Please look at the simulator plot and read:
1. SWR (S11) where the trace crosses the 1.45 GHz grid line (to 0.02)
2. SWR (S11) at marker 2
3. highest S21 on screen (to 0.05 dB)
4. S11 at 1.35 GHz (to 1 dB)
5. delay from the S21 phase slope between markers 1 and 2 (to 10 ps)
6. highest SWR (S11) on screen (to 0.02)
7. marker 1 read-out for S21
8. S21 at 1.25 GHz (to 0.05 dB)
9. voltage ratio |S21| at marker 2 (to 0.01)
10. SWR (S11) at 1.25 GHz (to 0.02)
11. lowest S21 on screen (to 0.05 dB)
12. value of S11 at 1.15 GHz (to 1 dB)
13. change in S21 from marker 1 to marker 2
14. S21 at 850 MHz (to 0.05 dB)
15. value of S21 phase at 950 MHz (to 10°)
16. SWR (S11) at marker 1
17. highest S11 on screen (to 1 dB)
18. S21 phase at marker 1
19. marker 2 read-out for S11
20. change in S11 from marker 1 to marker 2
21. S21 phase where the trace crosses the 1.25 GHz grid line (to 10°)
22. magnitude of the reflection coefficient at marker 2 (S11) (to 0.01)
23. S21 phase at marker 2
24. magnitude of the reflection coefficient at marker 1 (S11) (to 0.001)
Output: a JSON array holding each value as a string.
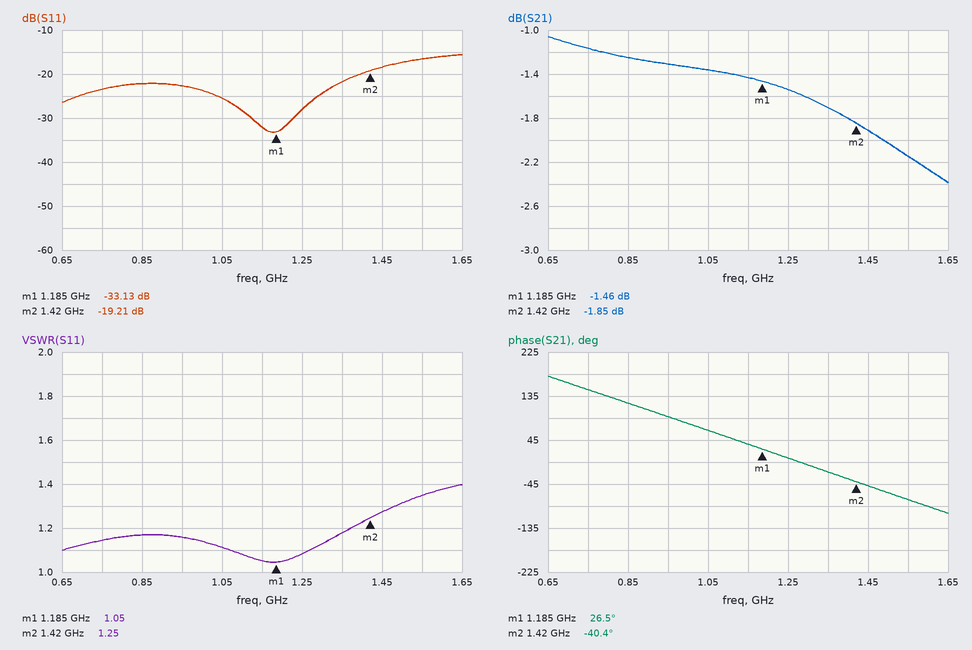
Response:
["1.28", "1.25", "-1.05 dB", "-22 dB", "790 ps", "1.40", "-1.46 dB", "-1.55 dB", "0.81", "1.08", "-2.40 dB", "-32 dB", "-0.39 dB", "-1.25 dB", "90°", "1.05", "-16 dB", "26.5°", "-19.21 dB", "13.92 dB", "10°", "0.11", "-40.4°", "0.022"]
